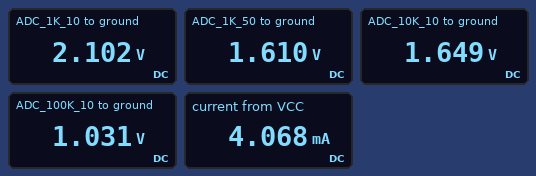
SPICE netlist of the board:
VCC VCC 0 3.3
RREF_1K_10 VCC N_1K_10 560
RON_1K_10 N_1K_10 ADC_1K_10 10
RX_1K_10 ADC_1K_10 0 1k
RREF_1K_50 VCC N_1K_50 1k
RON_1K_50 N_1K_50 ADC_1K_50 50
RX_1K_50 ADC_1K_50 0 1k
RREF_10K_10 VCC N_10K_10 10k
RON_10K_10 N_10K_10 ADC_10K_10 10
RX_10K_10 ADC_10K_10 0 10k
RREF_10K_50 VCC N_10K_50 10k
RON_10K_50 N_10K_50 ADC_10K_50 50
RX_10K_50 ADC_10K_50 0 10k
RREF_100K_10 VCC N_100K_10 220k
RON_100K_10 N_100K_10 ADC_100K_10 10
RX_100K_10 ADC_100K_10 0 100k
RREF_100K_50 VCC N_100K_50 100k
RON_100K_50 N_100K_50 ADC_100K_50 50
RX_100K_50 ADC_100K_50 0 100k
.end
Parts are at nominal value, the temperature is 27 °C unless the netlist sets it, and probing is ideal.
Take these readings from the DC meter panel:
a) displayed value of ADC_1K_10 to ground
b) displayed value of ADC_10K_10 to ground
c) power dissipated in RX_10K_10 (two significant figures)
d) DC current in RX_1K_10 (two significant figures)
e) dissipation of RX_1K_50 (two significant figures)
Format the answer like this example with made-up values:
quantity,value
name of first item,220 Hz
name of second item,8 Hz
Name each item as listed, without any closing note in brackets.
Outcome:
quantity,value
displayed value of ADC_1K_10 to ground,2.102 V
displayed value of ADC_10K_10 to ground,1.649 V
power dissipated in RX_10K_10,270 µW
DC current in RX_1K_10,2.1 mA
dissipation of RX_1K_50,2.6 mW
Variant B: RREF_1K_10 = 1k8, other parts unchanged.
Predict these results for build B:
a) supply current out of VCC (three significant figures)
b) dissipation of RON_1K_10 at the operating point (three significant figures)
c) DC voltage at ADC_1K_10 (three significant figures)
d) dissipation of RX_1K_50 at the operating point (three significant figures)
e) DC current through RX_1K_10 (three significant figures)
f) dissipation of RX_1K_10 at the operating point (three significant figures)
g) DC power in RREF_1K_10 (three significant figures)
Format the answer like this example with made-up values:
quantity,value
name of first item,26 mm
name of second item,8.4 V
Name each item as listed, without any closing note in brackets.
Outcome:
quantity,value
supply current out of VCC,3.14 mA
dissipation of RON_1K_10 at the operating point,13.8 µW
DC voltage at ADC_1K_10,1.17 V
dissipation of RX_1K_50 at the operating point,2.59 mW
DC current through RX_1K_10,1.17 mA
dissipation of RX_1K_10 at the operating point,1.38 mW
DC power in RREF_1K_10,2.48 mW
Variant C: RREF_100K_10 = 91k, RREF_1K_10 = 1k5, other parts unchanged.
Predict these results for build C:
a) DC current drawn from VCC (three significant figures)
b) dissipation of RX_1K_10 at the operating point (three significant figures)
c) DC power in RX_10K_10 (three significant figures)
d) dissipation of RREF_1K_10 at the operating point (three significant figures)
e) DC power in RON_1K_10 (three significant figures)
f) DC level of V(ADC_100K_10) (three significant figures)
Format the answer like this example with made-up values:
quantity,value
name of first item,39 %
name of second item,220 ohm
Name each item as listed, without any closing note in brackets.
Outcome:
quantity,value
DC current drawn from VCC,3.29 mA
dissipation of RX_1K_10 at the operating point,1.73 mW
DC power in RX_10K_10,272 µW
dissipation of RREF_1K_10 at the operating point,2.59 mW
DC power in RON_1K_10,17.3 µW
DC level of V(ADC_100K_10),1.73 V
